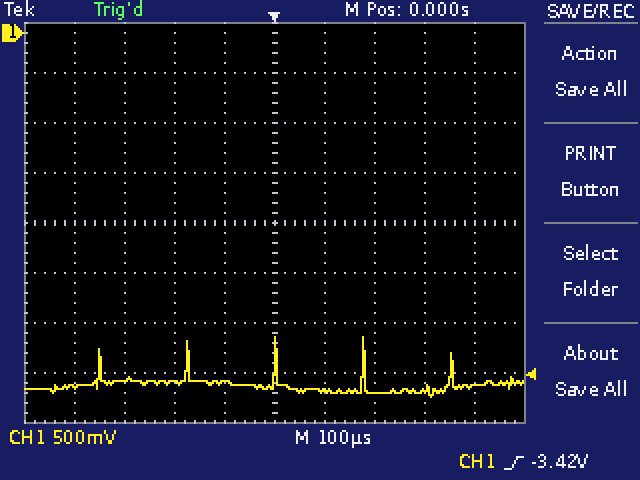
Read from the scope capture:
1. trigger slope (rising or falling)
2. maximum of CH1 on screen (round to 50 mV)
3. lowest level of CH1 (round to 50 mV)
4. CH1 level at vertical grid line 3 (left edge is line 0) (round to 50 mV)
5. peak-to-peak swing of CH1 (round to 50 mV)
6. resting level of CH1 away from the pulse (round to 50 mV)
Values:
rising
-3.05 V
-3.65 V
-3.50 V
600 mV
-3.50 V
